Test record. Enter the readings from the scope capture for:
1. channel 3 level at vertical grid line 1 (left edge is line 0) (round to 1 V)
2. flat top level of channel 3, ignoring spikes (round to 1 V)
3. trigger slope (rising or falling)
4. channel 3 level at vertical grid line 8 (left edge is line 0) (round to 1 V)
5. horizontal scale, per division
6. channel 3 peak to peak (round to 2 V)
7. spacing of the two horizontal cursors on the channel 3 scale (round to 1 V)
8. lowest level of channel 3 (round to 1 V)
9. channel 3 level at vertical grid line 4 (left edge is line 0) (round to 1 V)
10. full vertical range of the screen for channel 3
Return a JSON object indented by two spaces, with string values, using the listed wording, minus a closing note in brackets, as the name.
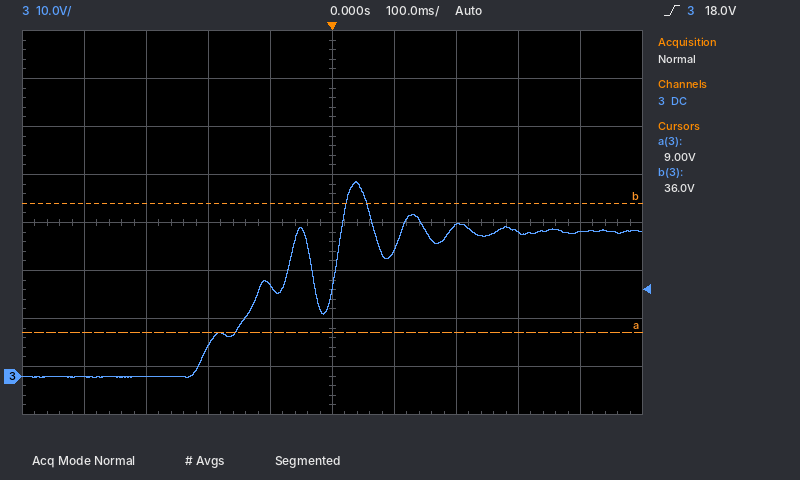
{
  "channel 3 level at vertical grid line 1 (left edge is line 0)": "0 V",
  "flat top level of channel 3, ignoring spikes": "30 V",
  "trigger slope": "rising",
  "channel 3 level at vertical grid line 8 (left edge is line 0)": "30 V",
  "horizontal scale, per division": "100 ms",
  "channel 3 peak to peak": "40 V",
  "spacing of the two horizontal cursors on the channel 3 scale": "27 V",
  "lowest level of channel 3": "0 V",
  "channel 3 level at vertical grid line 4 (left edge is line 0)": "19 V",
  "full vertical range of the screen for channel 3": "80 V"
}
